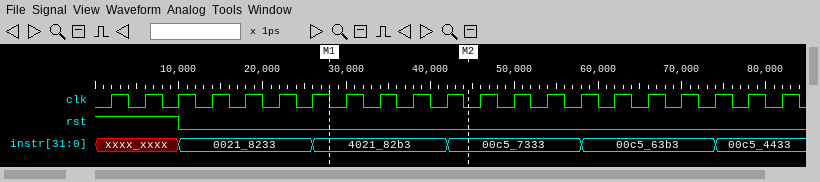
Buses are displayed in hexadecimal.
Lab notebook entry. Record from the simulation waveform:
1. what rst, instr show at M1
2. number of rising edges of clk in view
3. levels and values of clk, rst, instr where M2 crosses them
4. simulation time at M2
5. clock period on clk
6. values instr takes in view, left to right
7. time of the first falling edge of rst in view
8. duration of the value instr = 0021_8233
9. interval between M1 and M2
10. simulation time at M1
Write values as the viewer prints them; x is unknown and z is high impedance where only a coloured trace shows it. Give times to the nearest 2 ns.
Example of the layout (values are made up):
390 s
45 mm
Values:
rst=0, instr=4021_82b3
21
clk=0, rst=0, instr=00c5_7333
44 ns
4 ns
xxxx_xxxx, 0021_8233, 4021_82b3, 00c5_7333, 00c5_63b3, 00c5_4433
10 ns
16 ns
16 ns
28 ns
